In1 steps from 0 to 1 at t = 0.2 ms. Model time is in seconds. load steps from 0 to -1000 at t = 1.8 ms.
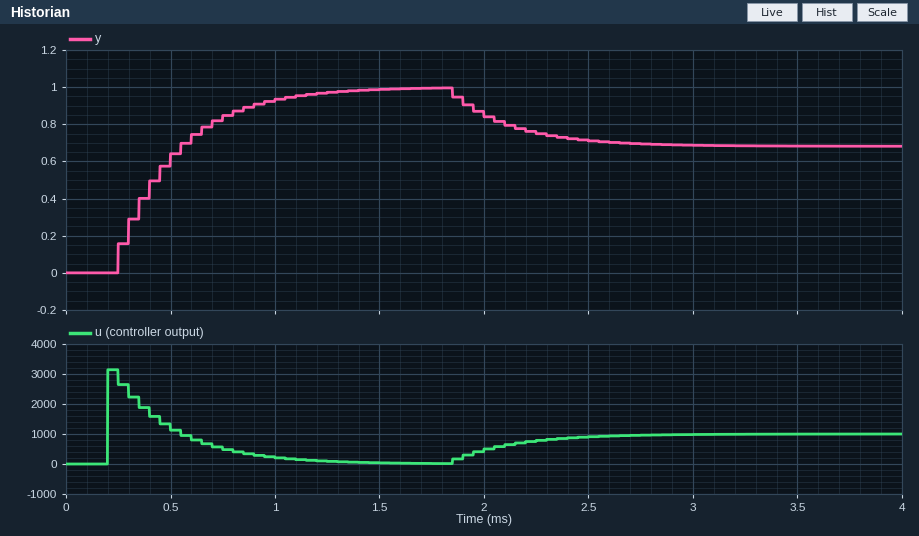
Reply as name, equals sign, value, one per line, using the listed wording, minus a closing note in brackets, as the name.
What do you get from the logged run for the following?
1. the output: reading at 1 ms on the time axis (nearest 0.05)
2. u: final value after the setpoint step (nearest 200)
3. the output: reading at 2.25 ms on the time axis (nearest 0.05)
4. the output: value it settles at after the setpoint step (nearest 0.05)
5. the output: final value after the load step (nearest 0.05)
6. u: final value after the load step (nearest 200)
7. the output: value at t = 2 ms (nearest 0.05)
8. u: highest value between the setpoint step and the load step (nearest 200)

the output: reading at 1 ms on the time axis = 0.95
u: final value after the setpoint step = 0
the output: reading at 2.25 ms on the time axis = 0.75
the output: value it settles at after the setpoint step = 1.00
the output: final value after the load step = 0.70
u: final value after the load step = 1000
the output: value at t = 2 ms = 0.85
u: highest value between the setpoint step and the load step = 3200
